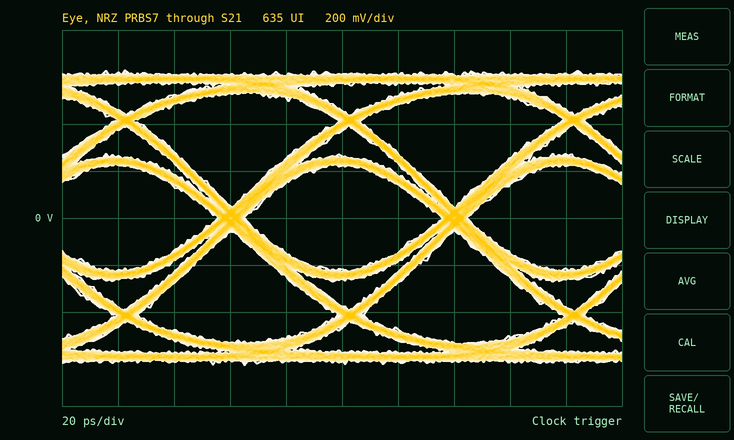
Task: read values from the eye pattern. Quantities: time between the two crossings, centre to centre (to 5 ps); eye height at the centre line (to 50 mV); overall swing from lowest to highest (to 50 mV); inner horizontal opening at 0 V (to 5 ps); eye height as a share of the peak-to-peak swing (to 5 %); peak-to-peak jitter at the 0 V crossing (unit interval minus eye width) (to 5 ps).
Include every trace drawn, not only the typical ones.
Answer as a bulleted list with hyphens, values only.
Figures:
- 80 ps
- 450 mV
- 1.25 V
- 70 ps
- 35 %
- 10 ps
